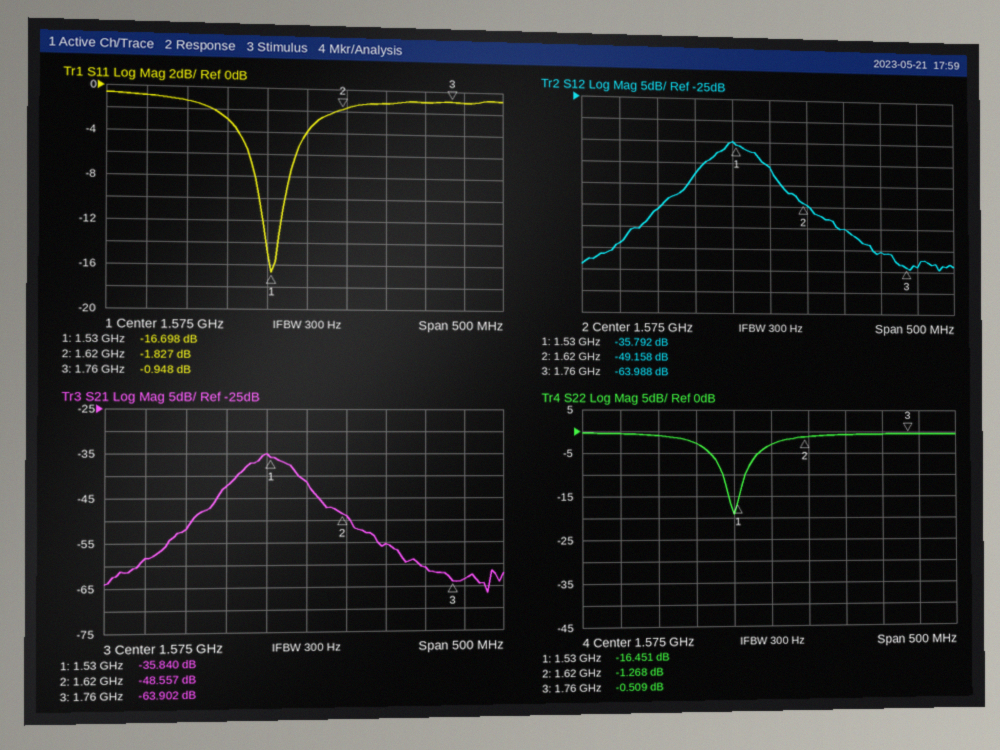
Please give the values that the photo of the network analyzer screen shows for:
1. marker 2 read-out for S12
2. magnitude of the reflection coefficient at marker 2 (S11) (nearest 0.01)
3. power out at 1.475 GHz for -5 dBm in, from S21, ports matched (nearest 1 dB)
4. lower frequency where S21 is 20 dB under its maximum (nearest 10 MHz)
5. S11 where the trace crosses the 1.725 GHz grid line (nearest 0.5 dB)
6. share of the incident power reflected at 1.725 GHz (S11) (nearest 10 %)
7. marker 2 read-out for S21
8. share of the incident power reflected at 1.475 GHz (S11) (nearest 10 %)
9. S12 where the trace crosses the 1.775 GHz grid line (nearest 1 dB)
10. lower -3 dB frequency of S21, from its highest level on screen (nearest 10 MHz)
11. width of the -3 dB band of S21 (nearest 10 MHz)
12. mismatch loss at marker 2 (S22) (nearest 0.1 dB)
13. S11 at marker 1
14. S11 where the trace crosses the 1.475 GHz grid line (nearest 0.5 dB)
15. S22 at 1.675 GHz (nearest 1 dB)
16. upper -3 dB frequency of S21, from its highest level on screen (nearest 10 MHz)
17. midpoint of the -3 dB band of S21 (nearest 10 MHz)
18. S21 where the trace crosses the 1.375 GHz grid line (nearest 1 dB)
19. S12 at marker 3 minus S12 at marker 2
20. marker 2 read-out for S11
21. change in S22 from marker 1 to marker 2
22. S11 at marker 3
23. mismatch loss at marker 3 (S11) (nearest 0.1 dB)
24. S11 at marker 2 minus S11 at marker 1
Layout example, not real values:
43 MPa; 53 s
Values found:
-49.158 dB; 0.81; -47 dBm; 1.40 GHz; -1.0 dB; 80 %; -48.557 dB; 50 %; -64 dB; 1.50 GHz; 60 MHz; 6.0 dB; -16.698 dB; -3.0 dB; -1 dB; 1.56 GHz; 1.53 GHz; -58 dB; -14.830 dB; -1.827 dB; 15.183 dB; -0.948 dB; 7.1 dB; 14.871 dB
